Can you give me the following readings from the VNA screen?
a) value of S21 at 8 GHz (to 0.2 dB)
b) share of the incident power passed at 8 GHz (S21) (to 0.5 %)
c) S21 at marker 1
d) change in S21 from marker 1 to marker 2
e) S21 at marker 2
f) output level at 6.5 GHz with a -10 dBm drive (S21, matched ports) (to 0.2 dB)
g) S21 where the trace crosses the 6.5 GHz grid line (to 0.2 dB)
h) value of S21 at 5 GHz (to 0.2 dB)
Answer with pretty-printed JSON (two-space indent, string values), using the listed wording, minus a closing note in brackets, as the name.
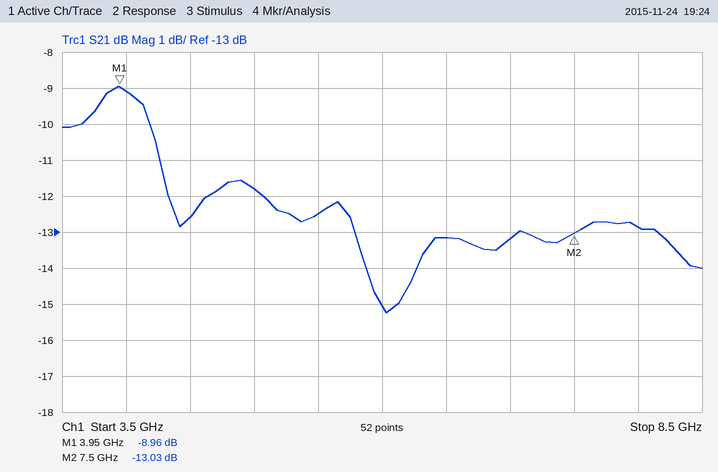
{
  "value of S21 at 8 GHz": "-12.8 dB",
  "share of the incident power passed at 8 GHz (S21)": "5.0 %",
  "S21 at marker 1": "-8.96 dB",
  "change in S21 from marker 1 to marker 2": "-4.07 dB",
  "S21 at marker 2": "-13.03 dB",
  "output level at 6.5 GHz with a -10 dBm drive (S21, matched ports)": "-23.2 dBm",
  "S21 where the trace crosses the 6.5 GHz grid line": "-13.2 dB",
  "value of S21 at 5 GHz": "-11.8 dB"
}
